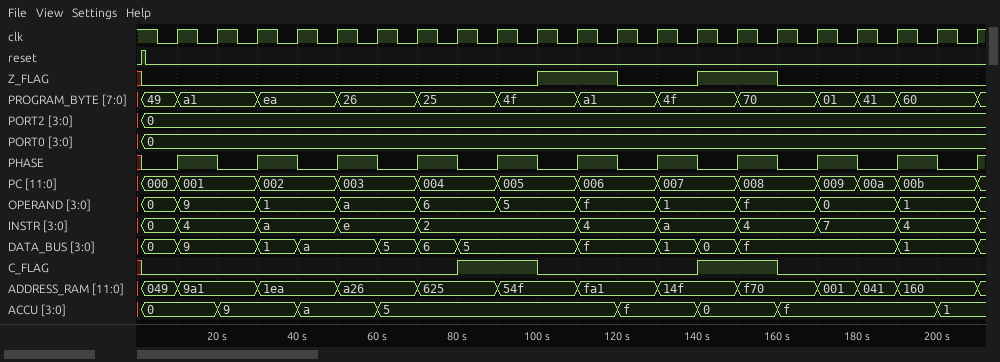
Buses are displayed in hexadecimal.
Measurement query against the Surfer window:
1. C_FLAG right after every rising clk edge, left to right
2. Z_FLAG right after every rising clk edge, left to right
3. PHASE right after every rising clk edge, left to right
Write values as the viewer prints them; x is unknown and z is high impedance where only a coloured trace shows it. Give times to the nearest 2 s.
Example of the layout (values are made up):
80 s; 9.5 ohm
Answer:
0 0 0 0 0 0 0 1 1 0 0 0 0 1 1 0 0 0 0 0 0; 0 0 0 0 0 0 0 0 0 1 1 0 0 1 1 0 0 0 0 0 0; 1 0 1 0 1 0 1 0 1 0 1 0 1 0 1 0 1 0 1 0 1
